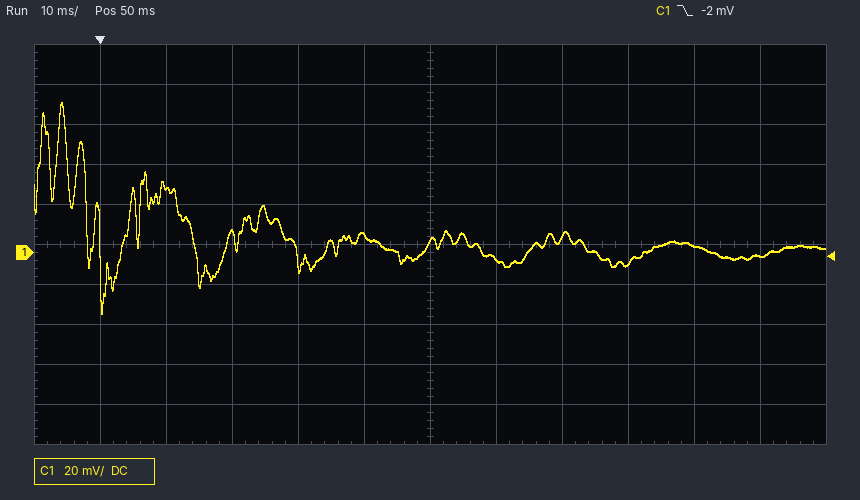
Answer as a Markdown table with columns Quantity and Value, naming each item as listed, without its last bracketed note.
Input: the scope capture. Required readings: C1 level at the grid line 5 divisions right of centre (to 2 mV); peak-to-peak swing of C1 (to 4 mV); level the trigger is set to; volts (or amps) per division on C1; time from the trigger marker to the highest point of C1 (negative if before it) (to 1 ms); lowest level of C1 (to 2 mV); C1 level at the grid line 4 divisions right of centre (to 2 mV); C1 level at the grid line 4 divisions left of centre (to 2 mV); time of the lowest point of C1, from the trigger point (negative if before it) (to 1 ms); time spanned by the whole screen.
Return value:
| Quantity | Value |
|---|---|
| C1 level at the grid line 5 divisions right of centre | -2 mV |
| peak-to-peak swing of C1 | 104 mV |
| level the trigger is set to | -2 mV |
| volts (or amps) per division on C1 | 20 mV |
| time from the trigger marker to the highest point of C1 (negative if before it) | -6 ms |
| lowest level of C1 | -30 mV |
| C1 level at the grid line 4 divisions right of centre | 4 mV |
| C1 level at the grid line 4 divisions left of centre | 34 mV |
| time of the lowest point of C1, from the trigger point (negative if before it) | 0 ms |
| time spanned by the whole screen | 120 ms |
